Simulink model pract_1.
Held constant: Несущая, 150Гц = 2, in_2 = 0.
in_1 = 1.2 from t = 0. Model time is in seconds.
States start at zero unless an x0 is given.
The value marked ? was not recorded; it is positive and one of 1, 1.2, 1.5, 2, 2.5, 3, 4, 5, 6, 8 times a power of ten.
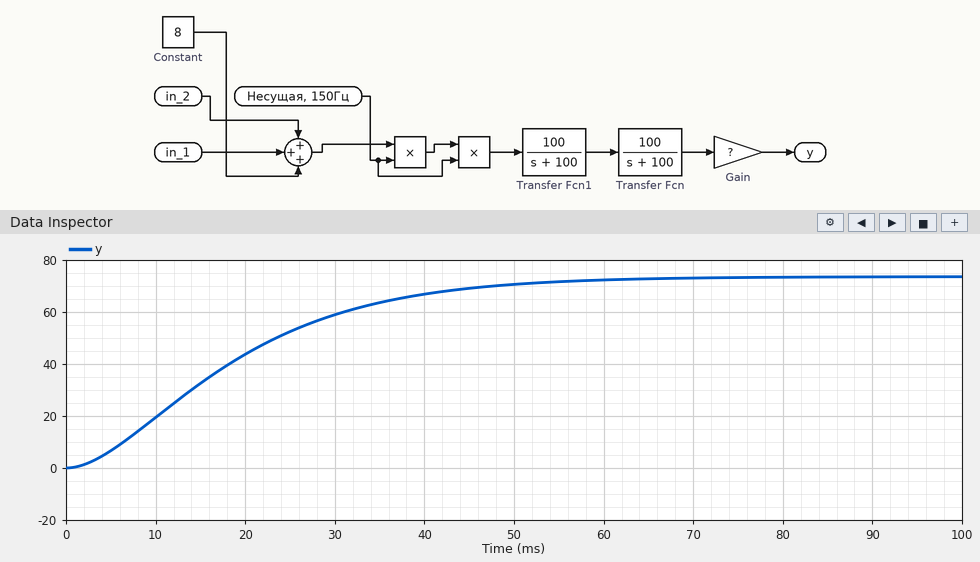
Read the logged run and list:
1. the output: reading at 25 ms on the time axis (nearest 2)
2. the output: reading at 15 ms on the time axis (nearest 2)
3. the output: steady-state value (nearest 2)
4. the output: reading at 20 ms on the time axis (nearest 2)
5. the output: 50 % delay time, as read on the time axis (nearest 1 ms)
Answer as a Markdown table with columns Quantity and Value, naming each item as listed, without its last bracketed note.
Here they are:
| Quantity | Value |
|---|---|
| the output: reading at 25 ms on the time axis | 52 |
| the output: reading at 15 ms on the time axis | 32 |
| the output: steady-state value | 74 |
| the output: reading at 20 ms on the time axis | 44 |
| the output: 50 % delay time, as read on the time axis | 17 ms |
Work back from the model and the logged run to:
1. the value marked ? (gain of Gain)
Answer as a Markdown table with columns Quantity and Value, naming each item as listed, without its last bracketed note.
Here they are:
| Quantity | Value |
|---|---|
| the value marked ? | 2 |
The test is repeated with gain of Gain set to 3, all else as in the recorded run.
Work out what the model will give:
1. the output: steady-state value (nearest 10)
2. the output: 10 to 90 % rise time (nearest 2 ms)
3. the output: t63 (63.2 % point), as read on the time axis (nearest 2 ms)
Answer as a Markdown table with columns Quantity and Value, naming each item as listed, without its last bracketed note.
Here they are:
| Quantity | Value |
|---|---|
| the output: steady-state value | 110 |
| the output: 10 to 90 % rise time | 34 ms |
| the output: t63 (63.2 % point), as read on the time axis | 22 ms |
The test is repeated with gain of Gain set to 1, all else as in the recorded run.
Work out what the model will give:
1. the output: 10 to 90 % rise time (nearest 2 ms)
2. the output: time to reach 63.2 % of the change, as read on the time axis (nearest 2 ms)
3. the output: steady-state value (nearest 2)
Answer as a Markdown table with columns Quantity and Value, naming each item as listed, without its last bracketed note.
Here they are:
| Quantity | Value |
|---|---|
| the output: 10 to 90 % rise time | 34 ms |
| the output: time to reach 63.2 % of the change, as read on the time axis | 22 ms |
| the output: steady-state value | 36 |
